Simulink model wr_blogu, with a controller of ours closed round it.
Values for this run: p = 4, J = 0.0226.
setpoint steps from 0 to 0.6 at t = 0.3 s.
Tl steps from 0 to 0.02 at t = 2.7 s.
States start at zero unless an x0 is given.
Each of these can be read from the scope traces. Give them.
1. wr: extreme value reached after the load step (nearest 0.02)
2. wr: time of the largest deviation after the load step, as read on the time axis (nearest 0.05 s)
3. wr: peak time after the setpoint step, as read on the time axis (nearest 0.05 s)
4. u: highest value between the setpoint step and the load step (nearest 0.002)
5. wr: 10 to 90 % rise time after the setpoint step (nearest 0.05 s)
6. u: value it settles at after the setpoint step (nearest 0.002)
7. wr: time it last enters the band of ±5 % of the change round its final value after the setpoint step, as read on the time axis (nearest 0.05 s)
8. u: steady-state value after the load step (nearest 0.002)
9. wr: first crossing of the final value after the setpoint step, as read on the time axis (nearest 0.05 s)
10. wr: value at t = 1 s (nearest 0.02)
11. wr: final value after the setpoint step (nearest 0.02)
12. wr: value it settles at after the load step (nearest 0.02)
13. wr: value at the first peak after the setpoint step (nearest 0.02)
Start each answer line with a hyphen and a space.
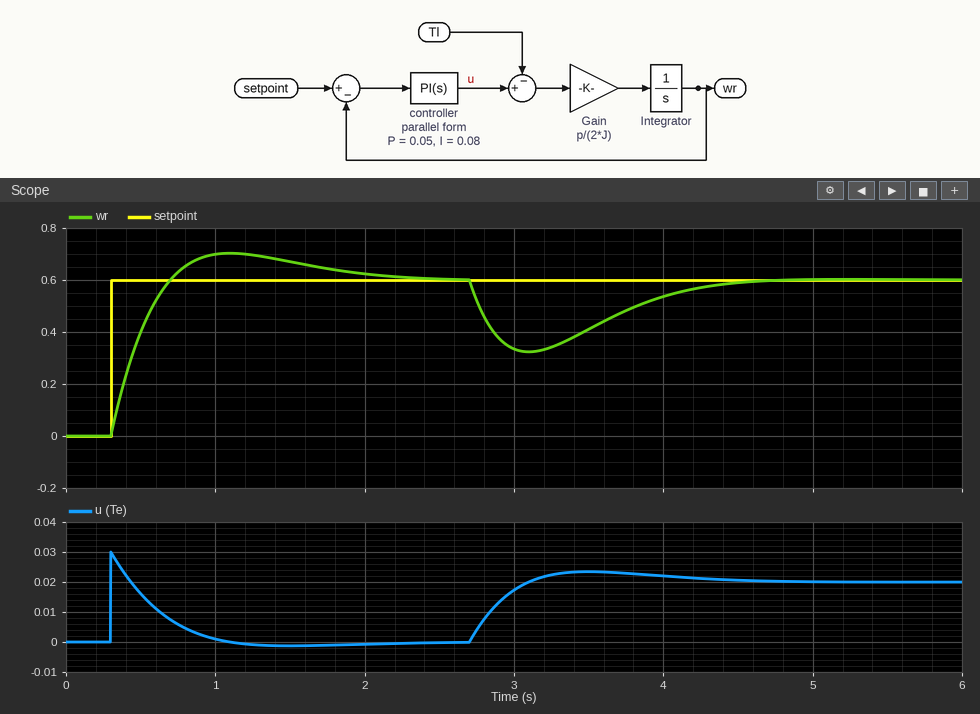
- 0.32
- 3.10 s
- 1.10 s
- 0.030
- 0.30 s
- 0.000
- 1.90 s
- 0.020
- 0.70 s
- 0.70
- 0.60
- 0.60
- 0.70
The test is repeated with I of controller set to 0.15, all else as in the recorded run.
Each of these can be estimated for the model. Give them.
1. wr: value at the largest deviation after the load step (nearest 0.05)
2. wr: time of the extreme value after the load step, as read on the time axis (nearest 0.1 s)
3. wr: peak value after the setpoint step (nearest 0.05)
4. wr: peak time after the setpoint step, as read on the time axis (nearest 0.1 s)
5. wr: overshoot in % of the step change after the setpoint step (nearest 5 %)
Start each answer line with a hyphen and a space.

- 0.35
- 3.0 s
- 0.75
- 0.9 s
- 25 %
